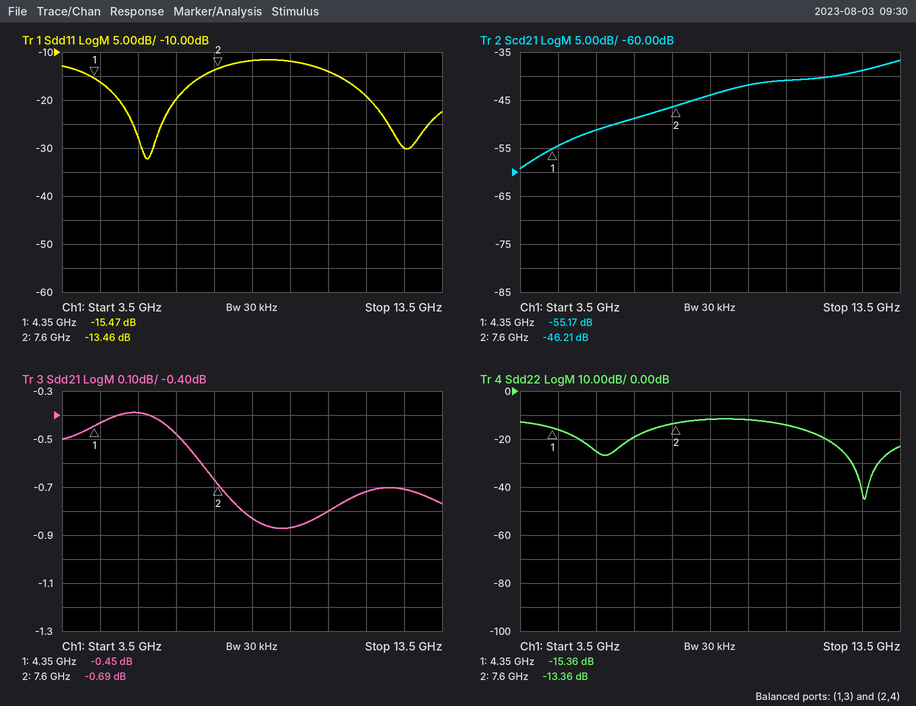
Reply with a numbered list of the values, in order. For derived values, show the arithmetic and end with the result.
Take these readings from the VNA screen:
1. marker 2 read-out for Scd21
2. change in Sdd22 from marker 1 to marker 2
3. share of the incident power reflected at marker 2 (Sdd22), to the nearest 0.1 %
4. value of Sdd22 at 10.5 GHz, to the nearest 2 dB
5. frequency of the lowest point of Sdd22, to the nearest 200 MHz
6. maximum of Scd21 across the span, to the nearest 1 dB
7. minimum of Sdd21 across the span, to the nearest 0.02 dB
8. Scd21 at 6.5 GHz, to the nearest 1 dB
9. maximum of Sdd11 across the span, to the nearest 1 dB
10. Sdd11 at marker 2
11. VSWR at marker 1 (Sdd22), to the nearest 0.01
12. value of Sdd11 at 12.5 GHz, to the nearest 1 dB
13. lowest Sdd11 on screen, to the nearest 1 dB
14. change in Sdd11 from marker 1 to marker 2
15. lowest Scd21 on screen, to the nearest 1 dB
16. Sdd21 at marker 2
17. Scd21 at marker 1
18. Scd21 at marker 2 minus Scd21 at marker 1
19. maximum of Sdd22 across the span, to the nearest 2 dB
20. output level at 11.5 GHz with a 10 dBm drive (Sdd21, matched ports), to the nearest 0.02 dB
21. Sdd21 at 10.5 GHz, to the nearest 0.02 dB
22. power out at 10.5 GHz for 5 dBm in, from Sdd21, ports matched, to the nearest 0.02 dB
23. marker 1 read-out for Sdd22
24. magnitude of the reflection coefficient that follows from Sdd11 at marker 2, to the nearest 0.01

1. -46.21 dB
2. -13.36 − (-15.36) = 2.00 dB
3. 10^(-13.36/10) ≈ 4.6 %
4. -14 dB
5. 12.6 GHz
6. -37 dB
7. -0.88 dB
8. -49 dB
9. -12 dB
10. -13.46 dB
11. (1 + 0.1706)/(1 − 0.1706) ≈ 1.41
12. -30 dB
13. -32 dB
14. -13.46 − (-15.47) = 2.01 dB
15. -59 dB
16. -0.69 dB
17. -55.17 dB
18. -46.21 − (-55.17) = 8.96 dB
19. -12 dB
20. 10 dBm + (-0.72 dB) = 9.28 dBm
21. -0.80 dB
22. 5 dBm + (-0.80 dB) = 4.20 dBm
23. -15.36 dB
24. 10^(-13.46/20) ≈ 0.21
